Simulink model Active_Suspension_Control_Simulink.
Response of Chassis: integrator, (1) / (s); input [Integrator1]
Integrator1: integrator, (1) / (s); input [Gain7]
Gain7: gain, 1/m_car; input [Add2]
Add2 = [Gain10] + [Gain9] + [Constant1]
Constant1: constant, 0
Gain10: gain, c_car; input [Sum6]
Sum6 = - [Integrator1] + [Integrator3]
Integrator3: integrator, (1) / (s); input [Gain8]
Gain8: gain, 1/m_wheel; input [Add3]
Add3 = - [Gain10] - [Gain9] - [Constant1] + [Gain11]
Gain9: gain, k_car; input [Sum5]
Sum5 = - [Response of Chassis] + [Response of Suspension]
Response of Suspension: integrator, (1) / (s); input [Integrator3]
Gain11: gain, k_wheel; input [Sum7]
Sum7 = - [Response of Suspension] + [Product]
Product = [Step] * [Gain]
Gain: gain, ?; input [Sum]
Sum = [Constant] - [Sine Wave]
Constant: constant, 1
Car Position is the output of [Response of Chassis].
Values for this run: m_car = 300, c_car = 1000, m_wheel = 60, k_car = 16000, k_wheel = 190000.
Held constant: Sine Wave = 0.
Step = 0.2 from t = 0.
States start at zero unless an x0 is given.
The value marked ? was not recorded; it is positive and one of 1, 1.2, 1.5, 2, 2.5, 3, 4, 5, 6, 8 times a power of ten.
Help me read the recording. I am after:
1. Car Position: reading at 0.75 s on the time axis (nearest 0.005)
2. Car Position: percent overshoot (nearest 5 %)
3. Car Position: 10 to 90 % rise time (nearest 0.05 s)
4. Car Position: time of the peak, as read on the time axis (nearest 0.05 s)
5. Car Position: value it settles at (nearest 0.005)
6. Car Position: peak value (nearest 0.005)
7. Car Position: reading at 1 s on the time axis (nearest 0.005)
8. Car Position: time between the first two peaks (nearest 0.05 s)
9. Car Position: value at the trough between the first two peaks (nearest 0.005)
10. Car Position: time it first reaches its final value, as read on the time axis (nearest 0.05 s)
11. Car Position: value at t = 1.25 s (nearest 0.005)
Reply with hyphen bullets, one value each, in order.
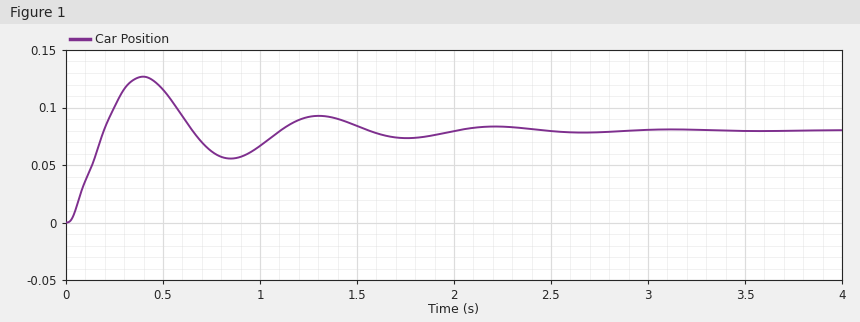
- 0.060
- 60 %
- 0.15 s
- 0.40 s
- 0.080
- 0.125
- 0.065
- 0.90 s
- 0.055
- 0.20 s
- 0.090
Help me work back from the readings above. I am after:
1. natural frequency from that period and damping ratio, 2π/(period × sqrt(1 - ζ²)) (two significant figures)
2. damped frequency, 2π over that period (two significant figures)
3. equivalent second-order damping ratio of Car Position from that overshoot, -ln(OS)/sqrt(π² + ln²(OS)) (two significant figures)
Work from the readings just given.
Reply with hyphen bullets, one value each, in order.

- 7.1 rad/s
- 7.0 rad/s
- 0.16
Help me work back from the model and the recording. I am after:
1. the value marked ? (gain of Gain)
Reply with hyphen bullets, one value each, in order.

- 0.4
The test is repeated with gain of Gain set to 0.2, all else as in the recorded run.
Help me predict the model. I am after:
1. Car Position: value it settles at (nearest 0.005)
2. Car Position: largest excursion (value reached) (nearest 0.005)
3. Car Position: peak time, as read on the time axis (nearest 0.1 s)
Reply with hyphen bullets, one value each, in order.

- 0.040
- 0.065
- 0.4 s
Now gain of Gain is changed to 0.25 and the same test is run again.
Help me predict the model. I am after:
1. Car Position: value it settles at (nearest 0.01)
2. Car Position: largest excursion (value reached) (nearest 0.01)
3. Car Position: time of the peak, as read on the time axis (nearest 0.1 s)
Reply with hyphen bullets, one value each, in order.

- 0.05
- 0.08
- 0.4 s
